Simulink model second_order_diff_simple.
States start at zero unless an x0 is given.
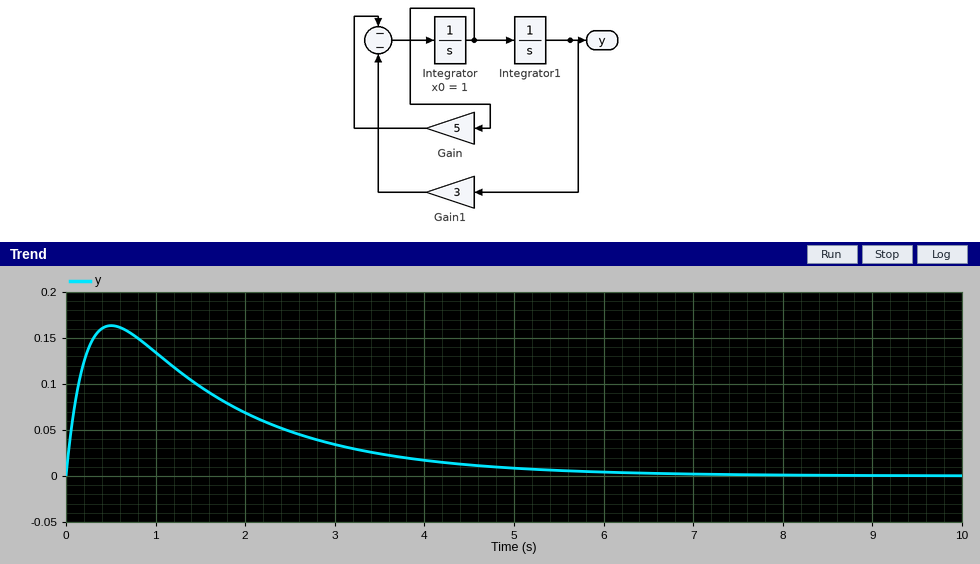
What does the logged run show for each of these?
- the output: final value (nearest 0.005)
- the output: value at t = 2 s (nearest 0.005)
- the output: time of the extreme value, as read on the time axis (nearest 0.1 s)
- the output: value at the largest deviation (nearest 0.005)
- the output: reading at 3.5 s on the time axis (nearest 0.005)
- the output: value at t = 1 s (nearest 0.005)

0.000
0.070
0.5 s
0.165
0.025
0.135
